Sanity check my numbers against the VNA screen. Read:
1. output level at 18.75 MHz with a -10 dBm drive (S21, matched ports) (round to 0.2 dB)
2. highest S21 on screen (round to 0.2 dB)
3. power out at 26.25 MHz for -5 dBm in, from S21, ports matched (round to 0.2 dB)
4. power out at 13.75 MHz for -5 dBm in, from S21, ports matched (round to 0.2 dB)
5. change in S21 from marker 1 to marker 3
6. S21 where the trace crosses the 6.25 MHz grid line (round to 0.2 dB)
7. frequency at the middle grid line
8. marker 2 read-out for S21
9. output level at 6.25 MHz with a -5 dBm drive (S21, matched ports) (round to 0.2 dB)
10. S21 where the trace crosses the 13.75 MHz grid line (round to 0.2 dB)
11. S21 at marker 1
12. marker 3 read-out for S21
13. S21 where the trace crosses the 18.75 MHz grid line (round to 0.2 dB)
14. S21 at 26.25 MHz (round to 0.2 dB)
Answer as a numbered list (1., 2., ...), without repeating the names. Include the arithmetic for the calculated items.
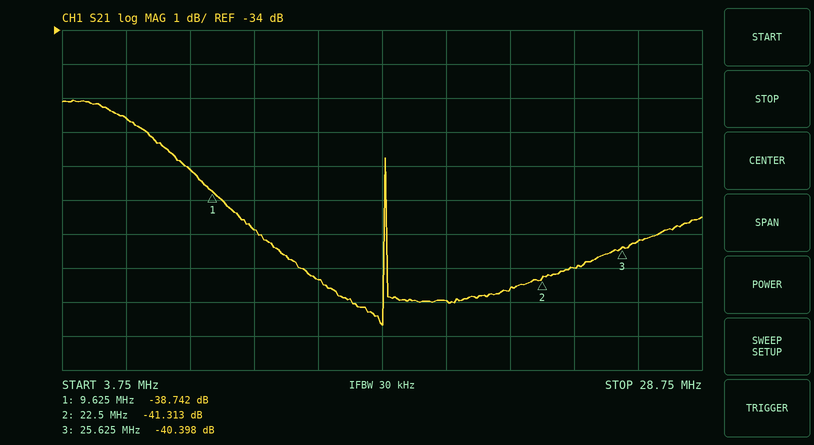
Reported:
1. -10 dBm + (-42.0 dB) = -52.0 dBm
2. -36.0 dB
3. -5 dBm + (-40.2 dB) = -45.2 dBm
4. -5 dBm + (-41.4 dB) = -46.4 dBm
5. -40.398 − (-38.742) = -1.656 dB
6. -36.6 dB
7. 16.25 MHz
8. -41.313 dB
9. -5 dBm + (-36.6 dB) = -41.6 dBm
10. -41.4 dB
11. -38.742 dB
12. -40.398 dB
13. -42.0 dB
14. -40.2 dB
